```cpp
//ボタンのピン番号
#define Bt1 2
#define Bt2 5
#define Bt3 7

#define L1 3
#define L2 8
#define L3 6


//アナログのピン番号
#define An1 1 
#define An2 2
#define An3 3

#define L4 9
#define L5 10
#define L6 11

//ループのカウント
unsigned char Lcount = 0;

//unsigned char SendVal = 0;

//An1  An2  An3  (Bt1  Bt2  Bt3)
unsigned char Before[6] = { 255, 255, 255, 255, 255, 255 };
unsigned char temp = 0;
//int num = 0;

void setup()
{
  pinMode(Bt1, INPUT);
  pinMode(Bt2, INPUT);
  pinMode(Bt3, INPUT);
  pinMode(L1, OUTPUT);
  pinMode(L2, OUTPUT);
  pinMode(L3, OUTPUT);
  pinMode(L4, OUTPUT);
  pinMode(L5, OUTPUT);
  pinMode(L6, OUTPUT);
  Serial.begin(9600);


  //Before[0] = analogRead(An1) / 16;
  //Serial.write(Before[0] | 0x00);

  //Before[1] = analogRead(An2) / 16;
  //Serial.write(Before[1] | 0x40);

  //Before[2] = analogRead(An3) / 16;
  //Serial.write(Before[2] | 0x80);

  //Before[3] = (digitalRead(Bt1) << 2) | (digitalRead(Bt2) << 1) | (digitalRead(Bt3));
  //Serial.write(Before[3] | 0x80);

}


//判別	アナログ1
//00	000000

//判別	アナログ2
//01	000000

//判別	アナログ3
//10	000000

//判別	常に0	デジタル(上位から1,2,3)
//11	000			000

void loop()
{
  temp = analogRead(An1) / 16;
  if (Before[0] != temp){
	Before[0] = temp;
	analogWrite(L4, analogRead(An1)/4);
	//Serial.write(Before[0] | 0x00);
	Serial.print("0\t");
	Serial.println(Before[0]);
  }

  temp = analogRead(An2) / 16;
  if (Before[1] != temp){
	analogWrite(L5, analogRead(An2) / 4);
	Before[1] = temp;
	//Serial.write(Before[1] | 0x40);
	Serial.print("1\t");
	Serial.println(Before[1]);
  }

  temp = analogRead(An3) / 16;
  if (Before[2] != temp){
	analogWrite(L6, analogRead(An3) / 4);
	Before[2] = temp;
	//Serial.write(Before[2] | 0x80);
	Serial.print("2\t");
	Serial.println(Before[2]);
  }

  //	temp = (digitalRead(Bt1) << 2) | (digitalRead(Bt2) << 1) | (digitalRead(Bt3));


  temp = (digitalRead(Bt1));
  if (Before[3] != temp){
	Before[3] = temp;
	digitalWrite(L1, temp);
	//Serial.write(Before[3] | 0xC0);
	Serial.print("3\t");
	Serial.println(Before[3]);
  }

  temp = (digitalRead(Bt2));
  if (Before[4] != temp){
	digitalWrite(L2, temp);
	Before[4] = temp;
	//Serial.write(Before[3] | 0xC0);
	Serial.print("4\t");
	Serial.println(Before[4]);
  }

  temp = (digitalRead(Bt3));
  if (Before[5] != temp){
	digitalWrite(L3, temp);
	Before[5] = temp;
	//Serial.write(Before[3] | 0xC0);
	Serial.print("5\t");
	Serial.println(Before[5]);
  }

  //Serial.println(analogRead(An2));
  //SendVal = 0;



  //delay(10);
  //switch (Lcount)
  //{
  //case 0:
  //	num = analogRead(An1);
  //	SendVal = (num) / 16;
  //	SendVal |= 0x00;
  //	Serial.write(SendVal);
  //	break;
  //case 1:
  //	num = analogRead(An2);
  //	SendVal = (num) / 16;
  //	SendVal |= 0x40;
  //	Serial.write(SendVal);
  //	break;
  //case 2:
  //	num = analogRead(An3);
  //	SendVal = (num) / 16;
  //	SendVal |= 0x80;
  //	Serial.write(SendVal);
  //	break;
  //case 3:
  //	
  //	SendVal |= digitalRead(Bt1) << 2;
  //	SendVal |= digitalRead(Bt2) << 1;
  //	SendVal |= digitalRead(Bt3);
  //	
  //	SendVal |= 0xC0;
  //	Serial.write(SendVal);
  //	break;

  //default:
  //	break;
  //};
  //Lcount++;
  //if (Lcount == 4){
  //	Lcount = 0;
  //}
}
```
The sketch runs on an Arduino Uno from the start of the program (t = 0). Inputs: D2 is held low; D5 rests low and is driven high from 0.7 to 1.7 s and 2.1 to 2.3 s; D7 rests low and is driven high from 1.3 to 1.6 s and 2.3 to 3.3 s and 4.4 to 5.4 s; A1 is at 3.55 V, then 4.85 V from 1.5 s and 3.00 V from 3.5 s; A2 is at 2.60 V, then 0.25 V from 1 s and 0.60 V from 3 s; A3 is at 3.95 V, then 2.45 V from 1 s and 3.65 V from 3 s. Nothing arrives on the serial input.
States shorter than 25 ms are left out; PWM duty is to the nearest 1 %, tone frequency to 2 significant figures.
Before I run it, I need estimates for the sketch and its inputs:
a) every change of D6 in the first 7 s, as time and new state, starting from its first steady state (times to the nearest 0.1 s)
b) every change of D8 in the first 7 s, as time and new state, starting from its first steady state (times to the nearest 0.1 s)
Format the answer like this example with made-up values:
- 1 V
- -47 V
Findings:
- 0 s low; 1.3 s high; 1.6 s low; 2.3 s high; 3.3 s low; 4.4 s high; 5.4 s low
- 0 s low; 0.7 s high; 1.7 s low; 2.1 s high; 2.3 s low
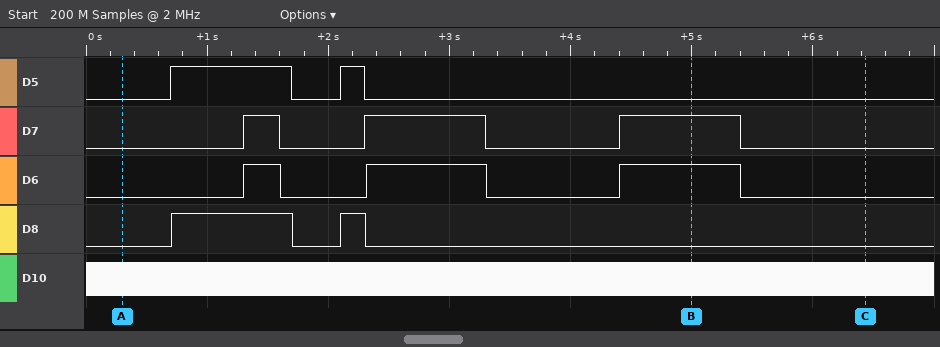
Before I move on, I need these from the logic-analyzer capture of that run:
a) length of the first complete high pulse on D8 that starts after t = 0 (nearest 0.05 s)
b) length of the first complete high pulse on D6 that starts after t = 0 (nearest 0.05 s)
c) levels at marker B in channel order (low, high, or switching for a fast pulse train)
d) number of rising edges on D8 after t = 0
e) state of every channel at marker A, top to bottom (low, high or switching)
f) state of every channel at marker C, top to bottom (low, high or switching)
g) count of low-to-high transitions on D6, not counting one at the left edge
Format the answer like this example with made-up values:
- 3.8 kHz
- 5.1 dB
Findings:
- 1.00 s
- 0.30 s
- D5 low, D7 high, D6 high, D8 low, D10 switching
- 2
- D5 low, D7 low, D6 low, D8 low, D10 switching
- D5 low, D7 low, D6 low, D8 low, D10 switching
- 3
